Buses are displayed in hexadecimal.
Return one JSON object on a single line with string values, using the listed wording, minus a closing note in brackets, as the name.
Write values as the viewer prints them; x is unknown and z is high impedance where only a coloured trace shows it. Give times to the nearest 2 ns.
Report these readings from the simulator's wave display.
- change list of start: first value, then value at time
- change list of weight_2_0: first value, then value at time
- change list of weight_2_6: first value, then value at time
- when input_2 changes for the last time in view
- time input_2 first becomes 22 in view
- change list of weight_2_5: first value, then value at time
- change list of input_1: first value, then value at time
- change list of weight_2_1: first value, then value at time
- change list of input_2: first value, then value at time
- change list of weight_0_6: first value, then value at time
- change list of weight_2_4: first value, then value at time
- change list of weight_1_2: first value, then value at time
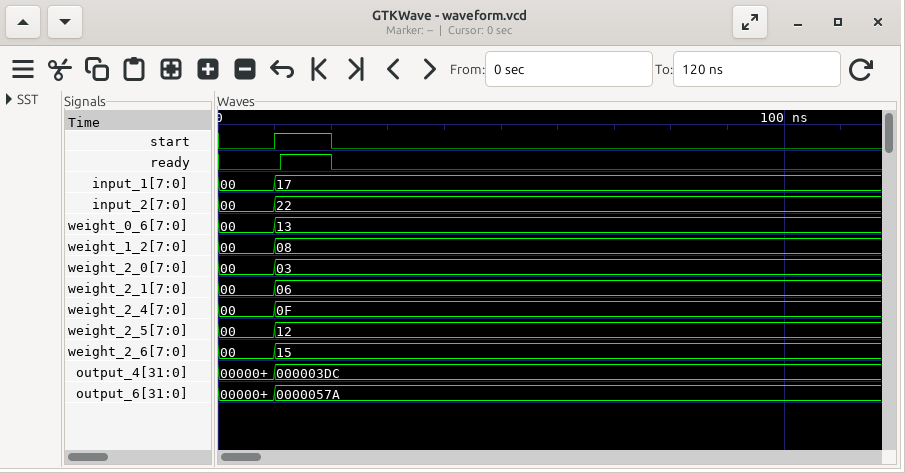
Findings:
{"change list of start: first value, then value at time": "0, 1 at 10 ns, 0 at 20 ns", "change list of weight_2_0: first value, then value at time": "00, 03 at 10 ns", "change list of weight_2_6: first value, then value at time": "00, 15 at 10 ns", "when input_2 changes for the last time in view": "10 ns", "time input_2 first becomes 22 in view": "10 ns", "change list of weight_2_5: first value, then value at time": "00, 12 at 10 ns", "change list of input_1: first value, then value at time": "00, 17 at 10 ns", "change list of weight_2_1: first value, then value at time": "00, 06 at 10 ns", "change list of input_2: first value, then value at time": "00, 22 at 10 ns", "change list of weight_0_6: first value, then value at time": "00, 13 at 10 ns", "change list of weight_2_4: first value, then value at time": "00, 0F at 10 ns", "change list of weight_1_2: first value, then value at time": "00, 08 at 10 ns"}
